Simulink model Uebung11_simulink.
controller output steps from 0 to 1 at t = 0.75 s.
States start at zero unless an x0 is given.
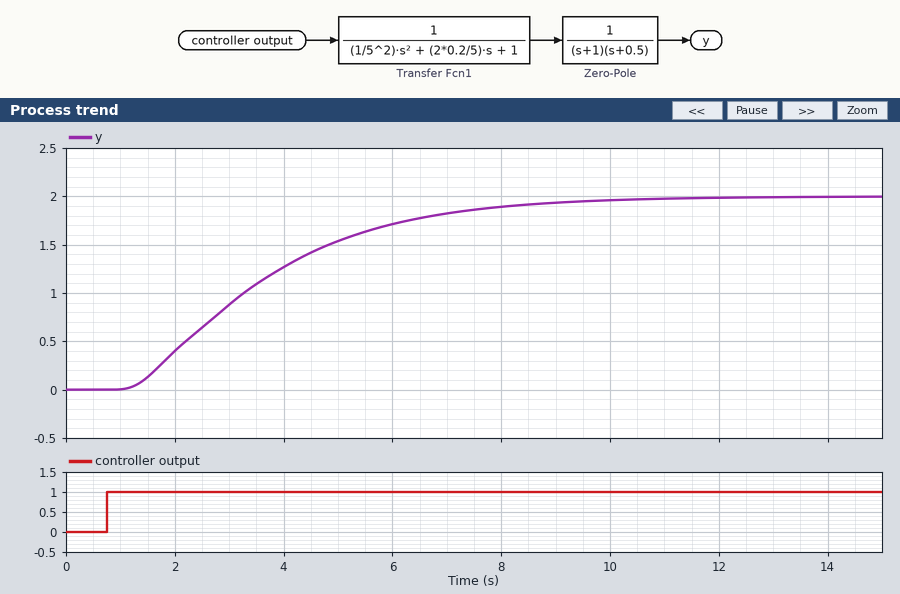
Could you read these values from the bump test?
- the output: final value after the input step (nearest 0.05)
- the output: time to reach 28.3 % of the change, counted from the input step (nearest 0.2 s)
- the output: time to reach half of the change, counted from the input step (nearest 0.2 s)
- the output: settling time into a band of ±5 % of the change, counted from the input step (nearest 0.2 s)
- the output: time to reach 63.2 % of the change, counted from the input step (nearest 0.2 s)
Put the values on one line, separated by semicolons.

2.00; 1.6 s; 2.6 s; 7.4 s; 3.2 s
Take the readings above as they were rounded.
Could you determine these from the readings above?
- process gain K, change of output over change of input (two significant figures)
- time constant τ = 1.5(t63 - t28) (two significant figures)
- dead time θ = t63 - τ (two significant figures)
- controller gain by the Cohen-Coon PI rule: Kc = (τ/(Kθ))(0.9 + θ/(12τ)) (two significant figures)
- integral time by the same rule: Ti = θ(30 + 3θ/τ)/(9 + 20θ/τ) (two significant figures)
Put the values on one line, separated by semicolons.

2.0; 2.4 s; 0.80 s; 1.4; 1.6 s
